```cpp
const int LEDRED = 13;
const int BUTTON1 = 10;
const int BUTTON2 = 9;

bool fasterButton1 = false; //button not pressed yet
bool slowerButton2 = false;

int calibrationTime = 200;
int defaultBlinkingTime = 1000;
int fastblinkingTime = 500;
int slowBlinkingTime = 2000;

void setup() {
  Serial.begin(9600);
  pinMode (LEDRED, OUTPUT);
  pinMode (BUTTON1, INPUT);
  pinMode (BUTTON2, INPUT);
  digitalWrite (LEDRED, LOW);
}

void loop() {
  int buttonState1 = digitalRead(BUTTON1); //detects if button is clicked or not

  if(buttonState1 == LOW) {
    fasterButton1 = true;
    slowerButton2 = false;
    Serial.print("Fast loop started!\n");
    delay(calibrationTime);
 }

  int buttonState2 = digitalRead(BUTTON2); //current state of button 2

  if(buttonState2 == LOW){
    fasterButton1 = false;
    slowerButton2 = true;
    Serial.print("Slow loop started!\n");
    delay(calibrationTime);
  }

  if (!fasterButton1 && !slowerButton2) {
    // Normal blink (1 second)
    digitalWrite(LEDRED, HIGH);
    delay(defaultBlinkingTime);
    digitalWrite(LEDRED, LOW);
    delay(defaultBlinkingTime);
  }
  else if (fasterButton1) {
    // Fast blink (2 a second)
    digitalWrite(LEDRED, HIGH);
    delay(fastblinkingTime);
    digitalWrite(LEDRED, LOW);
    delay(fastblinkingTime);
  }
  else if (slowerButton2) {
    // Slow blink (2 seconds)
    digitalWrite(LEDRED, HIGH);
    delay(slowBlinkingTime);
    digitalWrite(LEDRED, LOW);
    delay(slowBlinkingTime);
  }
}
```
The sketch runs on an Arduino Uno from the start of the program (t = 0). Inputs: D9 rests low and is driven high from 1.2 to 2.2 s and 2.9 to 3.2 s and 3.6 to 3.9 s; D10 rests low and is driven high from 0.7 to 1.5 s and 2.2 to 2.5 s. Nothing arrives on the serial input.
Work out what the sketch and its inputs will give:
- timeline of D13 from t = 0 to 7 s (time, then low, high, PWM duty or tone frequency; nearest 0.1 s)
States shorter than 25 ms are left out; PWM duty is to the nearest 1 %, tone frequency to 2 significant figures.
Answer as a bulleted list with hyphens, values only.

- 0 s low; 0.4 s high; 2.4 s low; 4.8 s high; 6.8 s low
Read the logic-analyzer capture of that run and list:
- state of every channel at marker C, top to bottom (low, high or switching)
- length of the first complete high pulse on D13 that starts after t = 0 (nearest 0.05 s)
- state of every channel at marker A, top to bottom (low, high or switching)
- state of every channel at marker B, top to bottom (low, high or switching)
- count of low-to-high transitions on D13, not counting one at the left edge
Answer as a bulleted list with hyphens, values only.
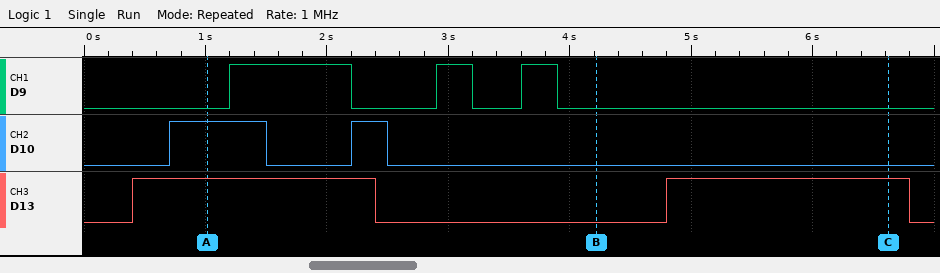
- D9 low, D10 low, D13 high
- 2.00 s
- D9 low, D10 high, D13 high
- D9 low, D10 low, D13 low
- 2
